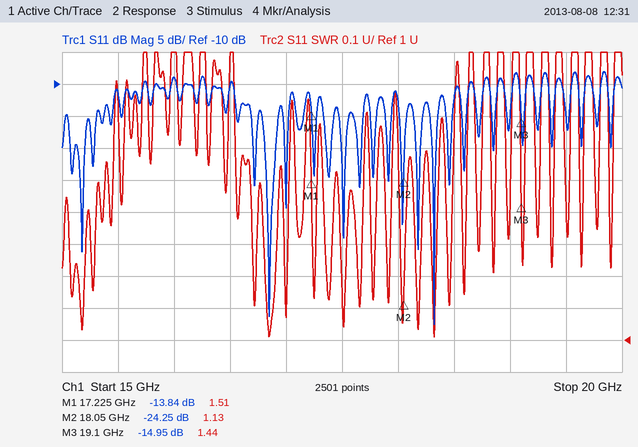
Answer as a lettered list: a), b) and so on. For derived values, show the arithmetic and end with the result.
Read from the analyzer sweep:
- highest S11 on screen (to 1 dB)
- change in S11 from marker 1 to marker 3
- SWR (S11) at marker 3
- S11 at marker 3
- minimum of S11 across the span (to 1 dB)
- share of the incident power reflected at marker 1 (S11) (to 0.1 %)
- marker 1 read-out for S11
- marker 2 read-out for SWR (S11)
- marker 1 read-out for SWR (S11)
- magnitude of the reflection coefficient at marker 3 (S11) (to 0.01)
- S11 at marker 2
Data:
a) -8 dB
b) -14.95 − (-13.84) = -1.11 dB
c) 1.44
d) -14.95 dB
e) -48 dB
f) 10^(-13.84/10) ≈ 4.1 %
g) -13.84 dB
h) 1.13
i) 1.51
j) 10^(-14.95/20) ≈ 0.18
k) -24.25 dB
